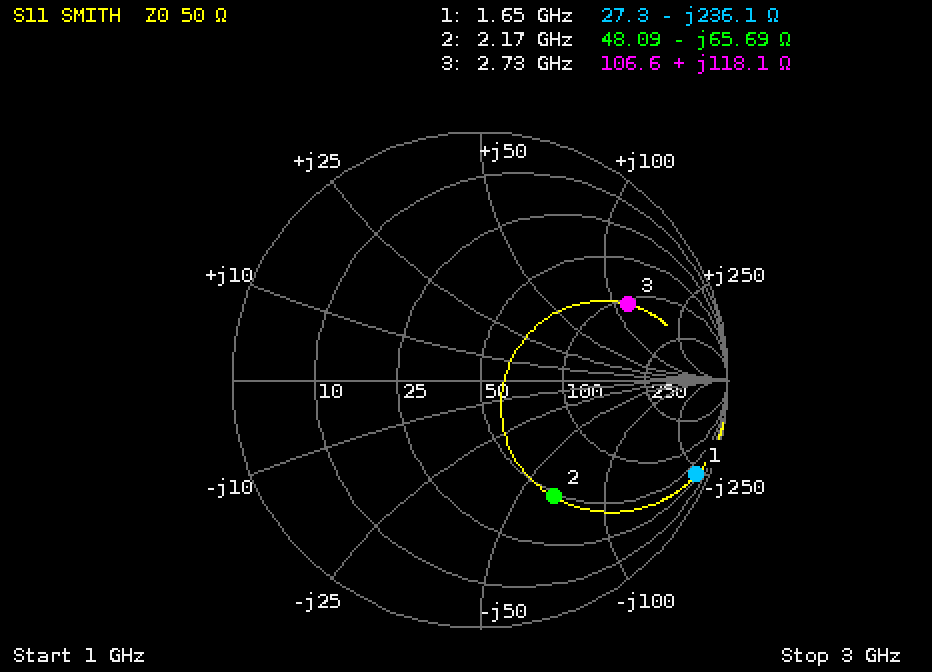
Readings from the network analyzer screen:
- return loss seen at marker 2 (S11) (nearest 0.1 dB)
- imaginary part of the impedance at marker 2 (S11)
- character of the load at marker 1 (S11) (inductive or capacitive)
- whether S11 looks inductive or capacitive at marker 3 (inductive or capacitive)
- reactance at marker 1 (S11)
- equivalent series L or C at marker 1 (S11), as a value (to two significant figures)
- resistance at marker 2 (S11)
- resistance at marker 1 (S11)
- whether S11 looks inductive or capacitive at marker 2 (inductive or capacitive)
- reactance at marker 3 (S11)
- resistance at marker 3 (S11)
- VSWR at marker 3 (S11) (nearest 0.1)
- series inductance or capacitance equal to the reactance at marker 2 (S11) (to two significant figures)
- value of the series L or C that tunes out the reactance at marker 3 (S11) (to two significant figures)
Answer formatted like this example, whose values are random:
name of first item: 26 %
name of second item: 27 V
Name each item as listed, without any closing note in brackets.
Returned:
return loss seen at marker 2 (S11): 5.1 dB
imaginary part of the impedance at marker 2: -65.69 Ω
character of the load at marker 1 (S11): capacitive
whether S11 looks inductive or capacitive at marker 3: inductive
reactance at marker 1: -236.1 Ω
equivalent series L or C at marker 1 (S11), as a value: 410 fF
resistance at marker 2: 48.09 Ω
resistance at marker 1: 27.3 Ω
whether S11 looks inductive or capacitive at marker 2: capacitive
reactance at marker 3: +118.1 Ω
resistance at marker 3: 106.6 Ω
VSWR at marker 3 (S11): 5.0
series inductance or capacitance equal to the reactance at marker 2 (S11): 1.1 pF
value of the series L or C that tunes out the reactance at marker 3 (S11): 490 fF
